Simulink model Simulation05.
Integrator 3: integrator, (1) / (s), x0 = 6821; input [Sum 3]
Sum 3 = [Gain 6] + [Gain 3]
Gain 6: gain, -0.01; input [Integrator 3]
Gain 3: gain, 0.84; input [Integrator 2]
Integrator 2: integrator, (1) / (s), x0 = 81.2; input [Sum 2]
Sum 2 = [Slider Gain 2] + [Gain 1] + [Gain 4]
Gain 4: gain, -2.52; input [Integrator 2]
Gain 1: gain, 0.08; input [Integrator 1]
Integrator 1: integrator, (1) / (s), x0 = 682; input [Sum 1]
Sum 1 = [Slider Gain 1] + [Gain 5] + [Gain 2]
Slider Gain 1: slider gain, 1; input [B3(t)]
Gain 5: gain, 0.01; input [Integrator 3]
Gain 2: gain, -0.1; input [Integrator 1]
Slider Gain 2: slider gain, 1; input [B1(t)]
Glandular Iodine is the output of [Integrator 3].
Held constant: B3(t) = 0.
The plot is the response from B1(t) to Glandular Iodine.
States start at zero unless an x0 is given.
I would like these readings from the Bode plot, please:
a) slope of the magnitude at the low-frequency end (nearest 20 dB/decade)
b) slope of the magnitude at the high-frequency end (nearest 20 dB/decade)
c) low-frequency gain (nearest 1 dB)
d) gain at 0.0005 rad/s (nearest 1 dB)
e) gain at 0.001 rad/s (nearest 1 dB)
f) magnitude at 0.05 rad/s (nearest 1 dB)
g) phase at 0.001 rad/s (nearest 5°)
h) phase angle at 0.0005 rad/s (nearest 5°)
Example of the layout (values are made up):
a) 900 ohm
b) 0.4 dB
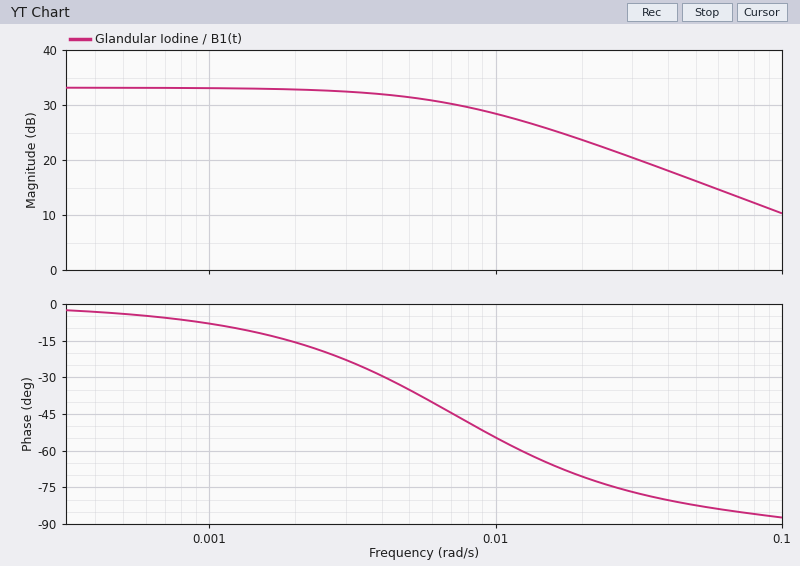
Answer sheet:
a) 0 dB/decade
b) -20 dB/decade
c) 33 dB
d) 33 dB
e) 33 dB
f) 16 dB
g) -10°
h) -5°
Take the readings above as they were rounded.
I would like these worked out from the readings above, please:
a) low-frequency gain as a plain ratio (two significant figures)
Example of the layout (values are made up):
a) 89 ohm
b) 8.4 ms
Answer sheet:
a) 45
